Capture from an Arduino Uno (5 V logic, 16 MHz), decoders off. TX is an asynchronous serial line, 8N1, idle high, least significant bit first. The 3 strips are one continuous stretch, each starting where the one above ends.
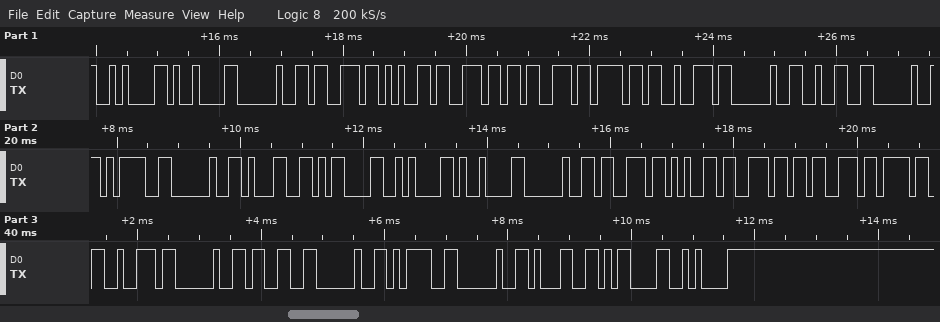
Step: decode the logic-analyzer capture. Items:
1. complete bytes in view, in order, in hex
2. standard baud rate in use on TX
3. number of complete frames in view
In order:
0A 09 20 73 65 6E 73 6F 72 20 32 20 3D 20 31 0D 0A 09 20 73 65 6E 73 6F 72 20 33 20 3D 20 31 0D 0A
9600 baud
33
